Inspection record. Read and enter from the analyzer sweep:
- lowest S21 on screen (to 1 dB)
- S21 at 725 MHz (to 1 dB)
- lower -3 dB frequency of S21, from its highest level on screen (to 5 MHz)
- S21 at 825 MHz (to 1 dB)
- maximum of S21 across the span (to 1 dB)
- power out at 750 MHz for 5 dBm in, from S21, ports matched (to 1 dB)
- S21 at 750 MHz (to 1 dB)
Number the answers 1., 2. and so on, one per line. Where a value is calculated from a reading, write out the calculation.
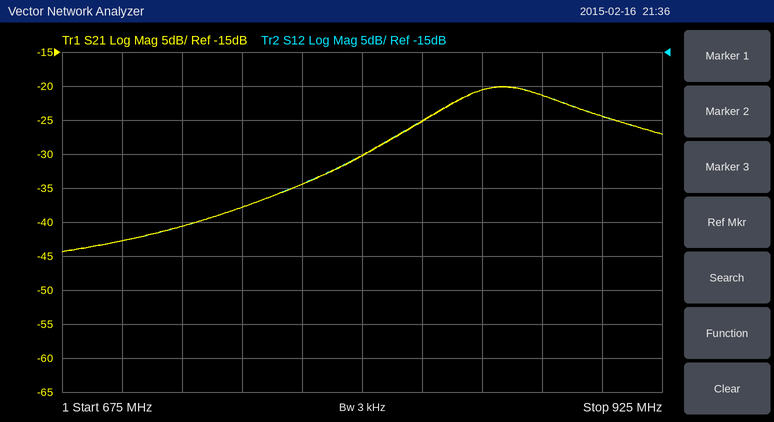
1. -44 dB
2. -41 dB
3. 835 MHz
4. -25 dB
5. -20 dB
6. 5 dBm + (-38 dB) = -33 dBm
7. -38 dB
